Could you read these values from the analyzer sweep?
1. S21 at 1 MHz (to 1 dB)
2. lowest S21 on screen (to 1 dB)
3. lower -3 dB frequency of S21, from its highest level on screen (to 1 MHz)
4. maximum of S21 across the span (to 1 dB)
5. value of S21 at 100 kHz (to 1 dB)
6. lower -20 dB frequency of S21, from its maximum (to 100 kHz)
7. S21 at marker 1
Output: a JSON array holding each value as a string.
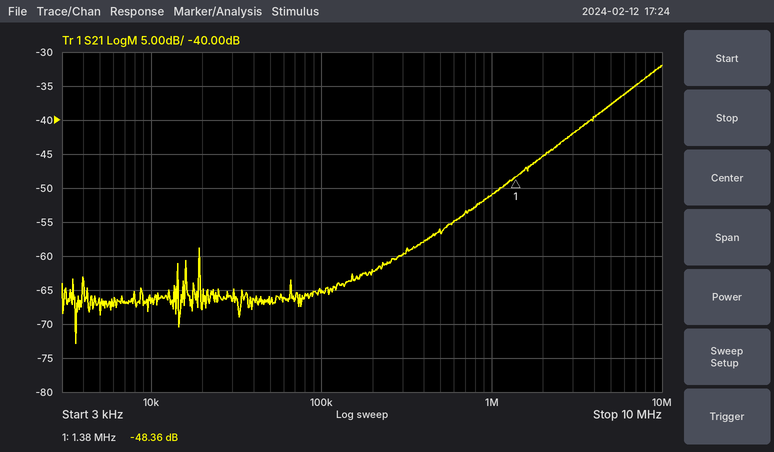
["-51 dB", "-73 dB", "7 MHz", "-32 dB", "-65 dB", "900 kHz", "-48.36 dB"]
